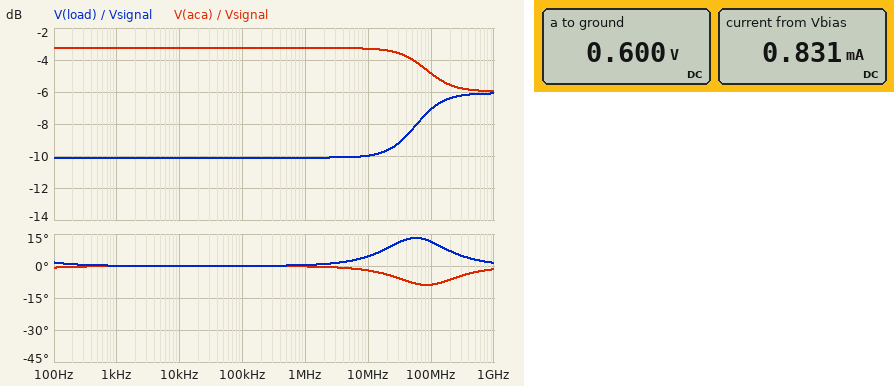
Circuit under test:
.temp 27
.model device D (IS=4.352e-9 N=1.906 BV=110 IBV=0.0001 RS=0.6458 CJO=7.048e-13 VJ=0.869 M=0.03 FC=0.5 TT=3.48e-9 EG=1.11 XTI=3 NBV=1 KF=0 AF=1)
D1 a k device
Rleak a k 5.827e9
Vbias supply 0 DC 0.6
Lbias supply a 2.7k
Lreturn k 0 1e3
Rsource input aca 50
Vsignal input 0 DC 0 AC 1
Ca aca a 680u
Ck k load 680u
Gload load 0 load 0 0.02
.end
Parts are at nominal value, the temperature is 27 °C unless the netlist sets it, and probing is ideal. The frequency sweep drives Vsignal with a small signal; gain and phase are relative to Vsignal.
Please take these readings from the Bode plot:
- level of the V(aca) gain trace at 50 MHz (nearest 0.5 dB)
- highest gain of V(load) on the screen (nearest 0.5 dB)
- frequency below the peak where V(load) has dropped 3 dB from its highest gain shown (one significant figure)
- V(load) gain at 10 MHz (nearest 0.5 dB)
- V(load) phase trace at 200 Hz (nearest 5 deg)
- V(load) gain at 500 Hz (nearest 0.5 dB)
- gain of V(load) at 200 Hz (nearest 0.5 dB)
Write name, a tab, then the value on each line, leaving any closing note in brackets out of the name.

level of the V(aca) gain trace at 50 MHz	-4.0 dB
highest gain of V(load) on the screen	-6.0 dB
frequency below the peak where V(load) has dropped 3 dB from its highest gain shown	30 MHz
V(load) gain at 10 MHz	-10.0 dB
V(load) phase trace at 200 Hz	0 deg
V(load) gain at 500 Hz	-10.0 dB
gain of V(load) at 200 Hz	-10.0 dB
